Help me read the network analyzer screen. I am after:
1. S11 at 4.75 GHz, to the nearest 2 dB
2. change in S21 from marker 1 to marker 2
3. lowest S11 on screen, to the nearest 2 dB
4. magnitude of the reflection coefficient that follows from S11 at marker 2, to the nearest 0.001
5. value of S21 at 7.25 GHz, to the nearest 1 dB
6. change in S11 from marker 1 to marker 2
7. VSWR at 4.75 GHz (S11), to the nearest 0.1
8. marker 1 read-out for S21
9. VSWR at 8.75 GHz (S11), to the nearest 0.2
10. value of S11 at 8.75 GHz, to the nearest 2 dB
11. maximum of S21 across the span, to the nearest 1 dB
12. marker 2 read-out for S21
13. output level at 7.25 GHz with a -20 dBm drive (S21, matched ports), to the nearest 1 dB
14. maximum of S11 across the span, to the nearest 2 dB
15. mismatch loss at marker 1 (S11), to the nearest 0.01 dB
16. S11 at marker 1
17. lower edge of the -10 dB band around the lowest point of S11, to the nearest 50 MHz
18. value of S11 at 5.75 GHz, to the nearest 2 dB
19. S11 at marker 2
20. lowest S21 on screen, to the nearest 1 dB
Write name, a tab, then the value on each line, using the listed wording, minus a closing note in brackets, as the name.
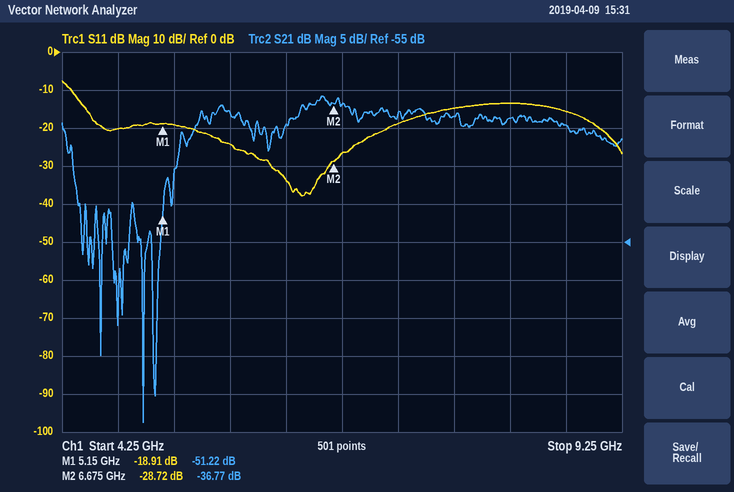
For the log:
S11 at 4.75 GHz, to the nearest 2 dB	-20 dB
change in S21 from marker 1 to marker 2	14.45 dB
lowest S11 on screen, to the nearest 2 dB	-38 dB
magnitude of the reflection coefficient that follows from S11 at marker 2, to the nearest 0.001	0.037
value of S21 at 7.25 GHz, to the nearest 1 dB	-38 dB
change in S11 from marker 1 to marker 2	-9.81 dB
VSWR at 4.75 GHz (S11), to the nearest 0.1	1.2
marker 1 read-out for S21	-51.22 dB
VSWR at 8.75 GHz (S11), to the nearest 0.2	1.4
value of S11 at 8.75 GHz, to the nearest 2 dB	-16 dB
maximum of S21 across the span, to the nearest 1 dB	-36 dB
marker 2 read-out for S21	-36.77 dB
output level at 7.25 GHz with a -20 dBm drive (S21, matched ports), to the nearest 1 dB	-58 dBm
maximum of S11 across the span, to the nearest 2 dB	-8 dB
mismatch loss at marker 1 (S11), to the nearest 0.01 dB	0.06 dB
S11 at marker 1	-18.91 dB
lower edge of the -10 dB band around the lowest point of S11, to the nearest 50 MHz	4.35 GHz
value of S11 at 5.75 GHz, to the nearest 2 dB	-24 dB
S11 at marker 2	-28.72 dB
lowest S21 on screen, to the nearest 1 dB	-79 dB
